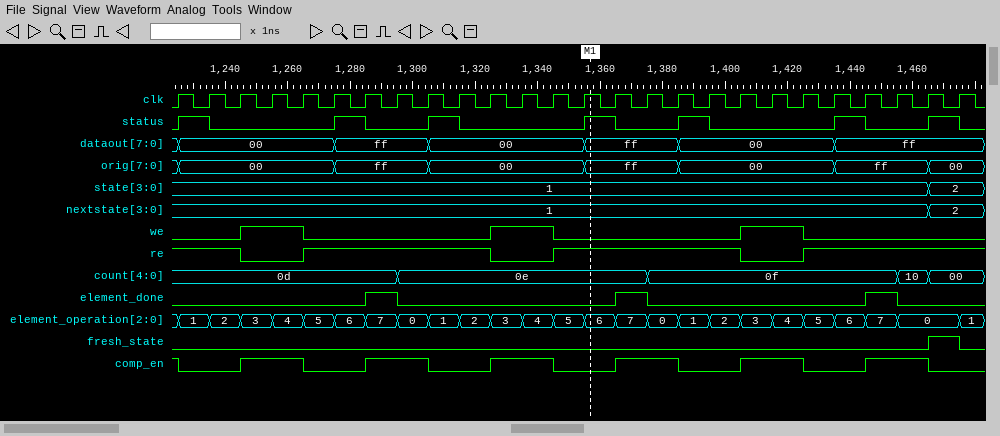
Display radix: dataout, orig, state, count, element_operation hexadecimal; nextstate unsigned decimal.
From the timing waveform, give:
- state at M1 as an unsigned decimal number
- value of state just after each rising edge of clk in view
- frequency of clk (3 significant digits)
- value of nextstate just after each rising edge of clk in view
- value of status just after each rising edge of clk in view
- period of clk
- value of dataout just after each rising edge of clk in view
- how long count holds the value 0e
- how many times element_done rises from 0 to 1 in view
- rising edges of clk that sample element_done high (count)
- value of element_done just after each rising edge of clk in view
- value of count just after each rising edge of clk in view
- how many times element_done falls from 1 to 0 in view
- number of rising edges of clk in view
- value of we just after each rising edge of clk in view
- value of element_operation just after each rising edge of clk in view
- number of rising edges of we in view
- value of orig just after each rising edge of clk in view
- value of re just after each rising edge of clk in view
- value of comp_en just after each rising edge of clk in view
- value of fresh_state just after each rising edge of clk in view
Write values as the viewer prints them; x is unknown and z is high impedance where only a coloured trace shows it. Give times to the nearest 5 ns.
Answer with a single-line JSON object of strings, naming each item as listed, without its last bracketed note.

{"state at M1 as an unsigned decimal number": "1", "value of state just after each rising edge of clk in view": "1, 1, 1, 1, 1, 1, 1, 1, 1, 1, 1, 1, 1, 1, 1, 1, 1, 1, 1, 1, 1, 1, 1, 1, 2, 2", "frequency of clk": "100 MHz", "value of nextstate just after each rising edge of clk in view": "1, 1, 1, 1, 1, 1, 1, 1, 1, 1, 1, 1, 1, 1, 1, 1, 1, 1, 1, 1, 1, 1, 1, 1, 2, 2", "value of status just after each rising edge of clk in view": "1 0 0 0 0 1 0 0 1 0 0 0 0 1 0 0 1 0 0 0 0 1 0 0 1 0", "period of clk": "10 ns", "value of dataout just after each rising edge of clk in view": "00, 00, 00, 00, 00, ff, ff, ff, 00, 00, 00, 00, 00, ff, ff, ff, 00, 00, 00, 00, 00, ff, ff, ff, ff, ff", "how long count holds the value 0e": "80 ns", "how many times element_done rises from 0 to 1 in view": "3", "rising edges of clk that sample element_done high": "3", "value of element_done just after each rising edge of clk in view": "0 0 0 0 0 0 1 0 0 0 0 0 0 0 1 0 0 0 0 0 0 0 1 0 0 0", "value of count just after each rising edge of clk in view": "0d, 0d, 0d, 0d, 0d, 0d, 0d, 0e, 0e, 0e, 0e, 0e, 0e, 0e, 0e, 0f, 0f, 0f, 0f, 0f, 0f, 0f, 0f, 10, 00, 00", "how many times element_done falls from 1 to 0 in view": "3", "number of rising edges of clk in view": "26", "value of we just after each rising edge of clk in view": "0 0 1 1 0 0 0 0 0 0 1 1 0 0 0 0 0 0 1 1 0 0 0 0 0 0", "value of element_operation just after each rising edge of clk in view": "1, 2, 3, 4, 5, 6, 7, 0, 1, 2, 3, 4, 5, 6, 7, 0, 1, 2, 3, 4, 5, 6, 7, 0, 0, 1", "number of rising edges of we in view": "3", "value of orig just after each rising edge of clk in view": "00, 00, 00, 00, 00, ff, ff, ff, 00, 00, 00, 00, 00, ff, ff, ff, 00, 00, 00, 00, 00, ff, ff, ff, 00, 00", "value of re just after each rising edge of clk in view": "1 1 0 0 1 1 1 1 1 1 0 0 1 1 1 1 1 1 0 0 1 1 1 1 1 1", "value of comp_en just after each rising edge of clk in view": "0 0 1 1 0 0 1 1 0 0 1 1 0 0 1 1 0 0 1 1 0 0 1 1 0 0", "value of fresh_state just after each rising edge of clk in view": "0 0 0 0 0 0 0 0 0 0 0 0 0 0 0 0 0 0 0 0 0 0 0 0 1 0"}
